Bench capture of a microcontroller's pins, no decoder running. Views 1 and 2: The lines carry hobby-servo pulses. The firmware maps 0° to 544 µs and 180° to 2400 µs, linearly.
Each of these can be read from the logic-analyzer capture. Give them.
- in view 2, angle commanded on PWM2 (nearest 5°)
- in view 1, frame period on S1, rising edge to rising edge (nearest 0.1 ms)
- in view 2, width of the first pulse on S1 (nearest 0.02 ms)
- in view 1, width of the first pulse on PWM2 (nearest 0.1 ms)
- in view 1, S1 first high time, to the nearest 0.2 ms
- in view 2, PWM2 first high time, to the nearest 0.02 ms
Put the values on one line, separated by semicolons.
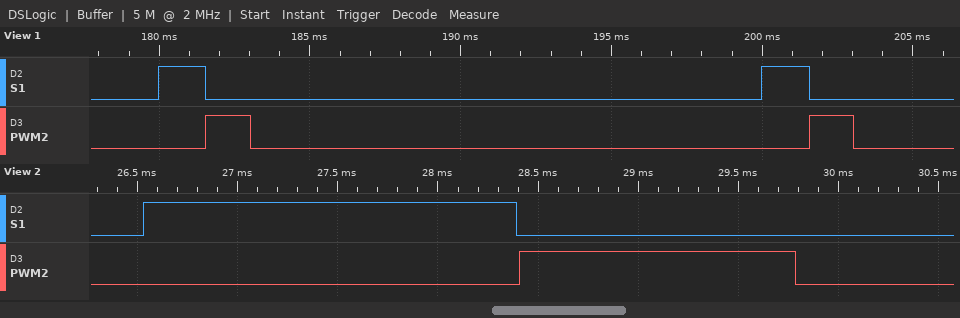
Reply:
80°; 20.0 ms; 1.86 ms; 1.5 ms; 1.6 ms; 1.38 ms
